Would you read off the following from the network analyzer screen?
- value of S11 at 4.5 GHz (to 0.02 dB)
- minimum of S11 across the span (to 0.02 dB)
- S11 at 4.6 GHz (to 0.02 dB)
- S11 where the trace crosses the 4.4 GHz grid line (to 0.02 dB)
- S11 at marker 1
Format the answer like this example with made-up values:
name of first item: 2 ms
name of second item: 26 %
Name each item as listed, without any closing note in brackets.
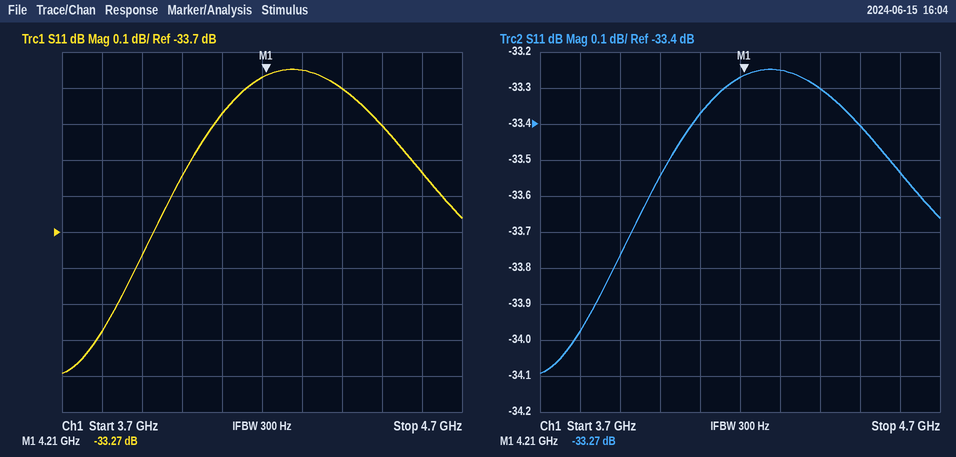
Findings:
value of S11 at 4.5 GHz: -33.40 dB
minimum of S11 across the span: -34.10 dB
S11 at 4.6 GHz: -33.54 dB
S11 where the trace crosses the 4.4 GHz grid line: -33.30 dB
S11 at marker 1: -33.27 dB
